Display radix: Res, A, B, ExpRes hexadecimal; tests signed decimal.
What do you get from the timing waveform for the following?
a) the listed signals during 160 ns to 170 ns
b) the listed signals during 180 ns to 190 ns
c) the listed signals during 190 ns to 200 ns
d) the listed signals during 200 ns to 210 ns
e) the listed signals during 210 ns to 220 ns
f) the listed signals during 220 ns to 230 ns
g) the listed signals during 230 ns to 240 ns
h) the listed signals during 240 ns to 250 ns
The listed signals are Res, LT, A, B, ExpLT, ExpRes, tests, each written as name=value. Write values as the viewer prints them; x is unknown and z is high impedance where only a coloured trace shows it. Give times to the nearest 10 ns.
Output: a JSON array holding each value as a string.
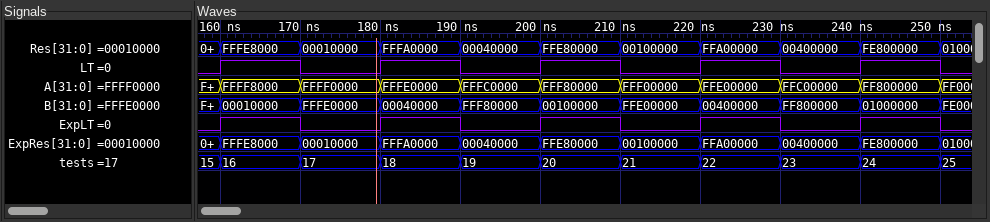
["Res=FFFE8000, LT=1, A=FFFF8000, B=00010000, ExpLT=1, ExpRes=FFFE8000, tests=16", "Res=FFFA0000, LT=1, A=FFFE0000, B=00040000, ExpLT=1, ExpRes=FFFA0000, tests=18", "Res=00040000, LT=0, A=FFFC0000, B=FFF80000, ExpLT=0, ExpRes=00040000, tests=19", "Res=FFE80000, LT=1, A=FFF80000, B=00100000, ExpLT=1, ExpRes=FFE80000, tests=20", "Res=00100000, LT=0, A=FFF00000, B=FFE00000, ExpLT=0, ExpRes=00100000, tests=21", "Res=FFA00000, LT=1, A=FFE00000, B=00400000, ExpLT=1, ExpRes=FFA00000, tests=22", "Res=00400000, LT=0, A=FFC00000, B=FF800000, ExpLT=0, ExpRes=00400000, tests=23", "Res=FE800000, LT=1, A=FF800000, B=01000000, ExpLT=1, ExpRes=FE800000, tests=24"]
